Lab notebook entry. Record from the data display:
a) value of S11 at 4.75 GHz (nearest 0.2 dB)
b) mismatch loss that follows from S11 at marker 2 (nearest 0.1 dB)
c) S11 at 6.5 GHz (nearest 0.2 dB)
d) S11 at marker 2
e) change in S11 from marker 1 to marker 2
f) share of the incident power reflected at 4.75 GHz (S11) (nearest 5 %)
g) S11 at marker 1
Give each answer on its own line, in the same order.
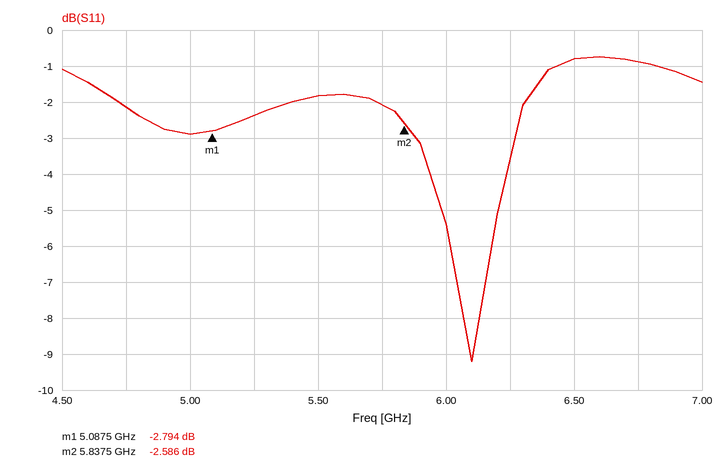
-2.2 dB
3.5 dB
-0.8 dB
-2.586 dB
0.208 dB
60 %
-2.794 dB
